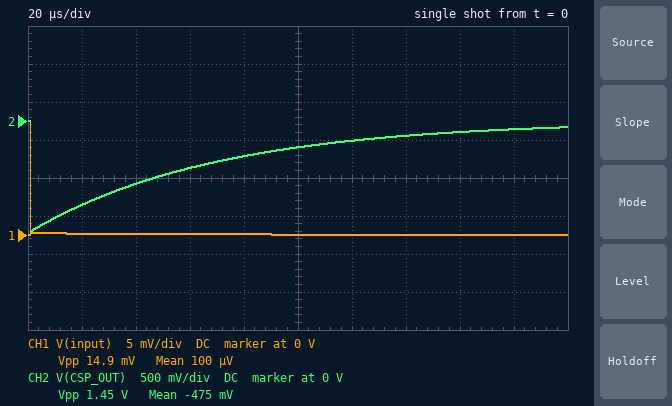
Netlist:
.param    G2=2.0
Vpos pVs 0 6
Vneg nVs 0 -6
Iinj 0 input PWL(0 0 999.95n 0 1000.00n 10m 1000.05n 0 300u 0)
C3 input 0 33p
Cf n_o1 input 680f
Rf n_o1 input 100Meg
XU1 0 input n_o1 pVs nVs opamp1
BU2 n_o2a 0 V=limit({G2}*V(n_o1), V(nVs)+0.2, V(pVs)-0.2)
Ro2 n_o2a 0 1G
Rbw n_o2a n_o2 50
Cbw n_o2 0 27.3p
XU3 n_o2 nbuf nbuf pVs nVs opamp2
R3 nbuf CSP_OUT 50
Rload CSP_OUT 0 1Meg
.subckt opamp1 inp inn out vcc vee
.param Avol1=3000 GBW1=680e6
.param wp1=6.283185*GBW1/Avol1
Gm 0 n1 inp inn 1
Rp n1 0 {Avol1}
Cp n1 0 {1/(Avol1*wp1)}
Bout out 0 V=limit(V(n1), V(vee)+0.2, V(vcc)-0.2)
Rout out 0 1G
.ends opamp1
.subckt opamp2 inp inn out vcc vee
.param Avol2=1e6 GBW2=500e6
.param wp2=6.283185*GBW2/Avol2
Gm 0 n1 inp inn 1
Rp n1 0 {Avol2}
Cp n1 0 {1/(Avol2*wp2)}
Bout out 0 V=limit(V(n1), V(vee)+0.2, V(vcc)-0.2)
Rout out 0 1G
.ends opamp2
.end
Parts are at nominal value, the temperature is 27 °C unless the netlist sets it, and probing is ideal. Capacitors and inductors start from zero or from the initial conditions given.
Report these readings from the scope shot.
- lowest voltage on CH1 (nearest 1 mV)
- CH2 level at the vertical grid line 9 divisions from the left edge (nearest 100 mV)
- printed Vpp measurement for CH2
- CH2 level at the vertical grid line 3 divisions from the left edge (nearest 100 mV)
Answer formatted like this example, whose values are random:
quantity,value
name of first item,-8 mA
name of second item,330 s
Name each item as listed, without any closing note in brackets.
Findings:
quantity,value
lowest voltage on CH1,0 V
CH2 level at the vertical grid line 9 divisions from the left edge,-100 mV
printed Vpp measurement for CH2,1.45 V
CH2 level at the vertical grid line 3 divisions from the left edge,-600 mV
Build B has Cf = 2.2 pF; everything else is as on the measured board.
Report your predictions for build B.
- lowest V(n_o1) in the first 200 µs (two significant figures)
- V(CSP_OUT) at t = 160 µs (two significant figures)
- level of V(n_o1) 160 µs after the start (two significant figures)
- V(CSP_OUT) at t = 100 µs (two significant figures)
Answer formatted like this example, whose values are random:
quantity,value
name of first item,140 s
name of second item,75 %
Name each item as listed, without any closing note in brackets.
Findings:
quantity,value
lowest V(n_o1) in the first 200 µs,-230 mV
V(CSP_OUT) at t = 160 µs,-220 mV
level of V(n_o1) 160 µs after the start,-110 mV
V(CSP_OUT) at t = 100 µs,-290 mV
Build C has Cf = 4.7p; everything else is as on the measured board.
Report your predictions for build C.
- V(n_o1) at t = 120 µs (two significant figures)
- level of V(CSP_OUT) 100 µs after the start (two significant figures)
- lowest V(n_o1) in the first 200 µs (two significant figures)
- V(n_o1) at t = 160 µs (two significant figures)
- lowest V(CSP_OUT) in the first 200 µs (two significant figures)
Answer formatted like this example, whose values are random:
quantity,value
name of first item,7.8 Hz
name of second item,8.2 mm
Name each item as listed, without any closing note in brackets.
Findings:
quantity,value
V(n_o1) at t = 120 µs,-83 mV
level of V(CSP_OUT) 100 µs after the start,-170 mV
lowest V(n_o1) in the first 200 µs,-110 mV
V(n_o1) at t = 160 µs,-76 mV
lowest V(CSP_OUT) in the first 200 µs,-210 mV
